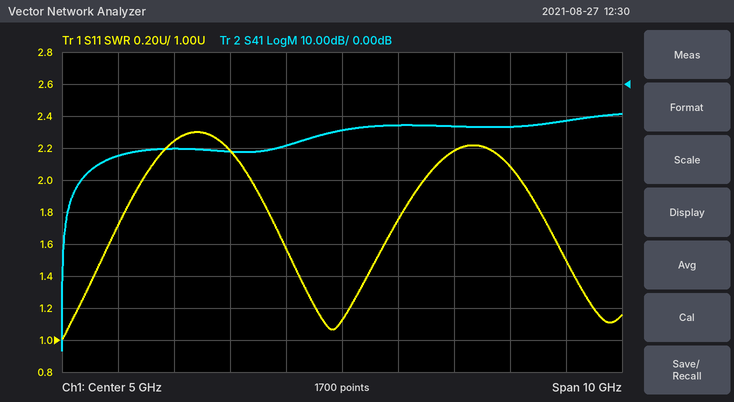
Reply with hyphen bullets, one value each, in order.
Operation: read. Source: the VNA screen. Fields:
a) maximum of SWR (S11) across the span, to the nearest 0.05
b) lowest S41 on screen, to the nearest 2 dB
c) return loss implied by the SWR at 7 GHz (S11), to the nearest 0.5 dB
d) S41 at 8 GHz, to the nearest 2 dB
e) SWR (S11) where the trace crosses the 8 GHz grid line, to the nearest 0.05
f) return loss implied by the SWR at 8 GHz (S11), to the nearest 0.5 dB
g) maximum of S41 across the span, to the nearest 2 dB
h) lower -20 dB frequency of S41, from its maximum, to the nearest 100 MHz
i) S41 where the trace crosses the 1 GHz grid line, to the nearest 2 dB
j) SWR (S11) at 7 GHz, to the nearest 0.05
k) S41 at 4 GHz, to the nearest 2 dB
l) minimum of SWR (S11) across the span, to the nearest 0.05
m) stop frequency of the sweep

- 2.30
- -84 dB
- 8.5 dB
- -14 dB
- 2.10
- 9.0 dB
- -10 dB
- 400 MHz
- -22 dB
- 2.20
- -20 dB
- 1.00
- 10 GHz
